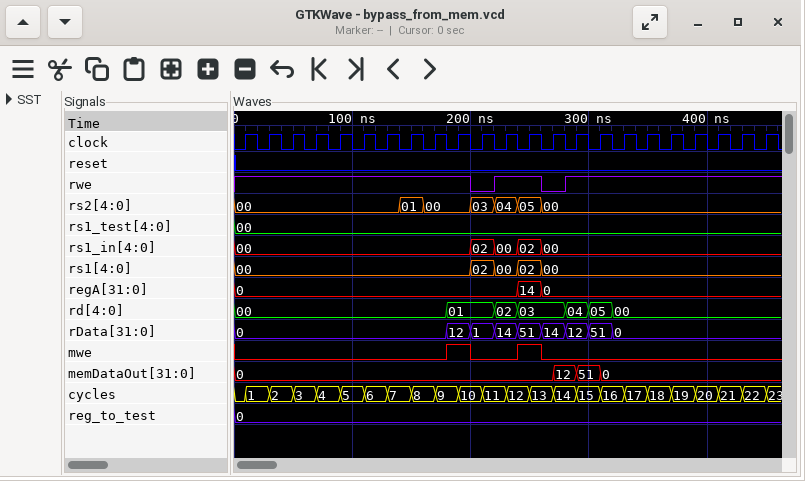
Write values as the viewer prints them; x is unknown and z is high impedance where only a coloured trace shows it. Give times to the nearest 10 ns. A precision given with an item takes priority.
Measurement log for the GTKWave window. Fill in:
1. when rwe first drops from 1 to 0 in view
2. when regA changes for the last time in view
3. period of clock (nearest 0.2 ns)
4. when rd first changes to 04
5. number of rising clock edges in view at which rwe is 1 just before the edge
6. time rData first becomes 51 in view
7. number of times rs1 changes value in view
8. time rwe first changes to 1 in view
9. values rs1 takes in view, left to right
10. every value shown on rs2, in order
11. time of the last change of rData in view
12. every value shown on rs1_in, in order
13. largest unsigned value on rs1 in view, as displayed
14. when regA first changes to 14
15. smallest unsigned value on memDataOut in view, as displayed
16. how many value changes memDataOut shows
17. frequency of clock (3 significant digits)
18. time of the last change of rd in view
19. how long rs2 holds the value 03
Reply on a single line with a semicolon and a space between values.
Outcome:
200 ns; 260 ns; 20 ns; 280 ns; 21; 240 ns; 4; 220 ns; 00, 02, 00, 02, 00; 00, 01, 00, 03, 04, 05, 00; 320 ns; 00, 02, 00, 02, 00; 02; 240 ns; 0; 3; 50.0 MHz; 320 ns; 20 ns
